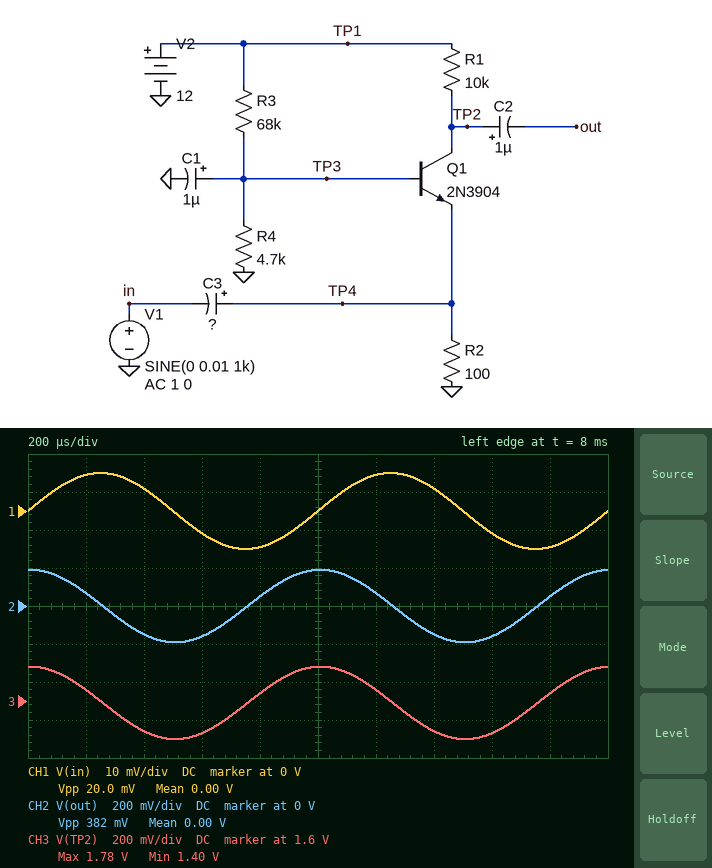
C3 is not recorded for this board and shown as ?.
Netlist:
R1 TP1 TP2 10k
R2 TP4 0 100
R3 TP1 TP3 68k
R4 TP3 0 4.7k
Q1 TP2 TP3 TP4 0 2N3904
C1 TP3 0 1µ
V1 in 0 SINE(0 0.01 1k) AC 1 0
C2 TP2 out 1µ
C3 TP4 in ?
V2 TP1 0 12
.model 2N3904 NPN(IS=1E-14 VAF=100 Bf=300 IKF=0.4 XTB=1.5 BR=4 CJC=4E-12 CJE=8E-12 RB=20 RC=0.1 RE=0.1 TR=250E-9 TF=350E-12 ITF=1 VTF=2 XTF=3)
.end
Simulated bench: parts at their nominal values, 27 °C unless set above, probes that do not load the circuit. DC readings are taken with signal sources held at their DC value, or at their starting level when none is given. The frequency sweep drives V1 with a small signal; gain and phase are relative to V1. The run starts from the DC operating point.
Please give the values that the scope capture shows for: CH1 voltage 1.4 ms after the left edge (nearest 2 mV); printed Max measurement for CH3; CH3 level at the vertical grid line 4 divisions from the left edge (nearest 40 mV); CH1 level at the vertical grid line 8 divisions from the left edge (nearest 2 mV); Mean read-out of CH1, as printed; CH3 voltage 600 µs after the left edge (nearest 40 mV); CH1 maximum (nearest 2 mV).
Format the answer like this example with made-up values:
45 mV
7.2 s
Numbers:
6 mV
1.78 V
1.64 V
-6 mV
0.00 V
1.44 V
10 mV
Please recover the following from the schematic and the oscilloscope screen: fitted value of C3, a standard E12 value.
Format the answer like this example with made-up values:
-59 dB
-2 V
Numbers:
390 nF
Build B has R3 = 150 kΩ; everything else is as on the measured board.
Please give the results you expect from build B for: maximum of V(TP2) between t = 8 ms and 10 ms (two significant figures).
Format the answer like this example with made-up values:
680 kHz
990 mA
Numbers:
12 V
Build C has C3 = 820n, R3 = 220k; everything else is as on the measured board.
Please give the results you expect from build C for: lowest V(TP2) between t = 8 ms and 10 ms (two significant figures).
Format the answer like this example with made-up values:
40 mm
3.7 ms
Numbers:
12 V
